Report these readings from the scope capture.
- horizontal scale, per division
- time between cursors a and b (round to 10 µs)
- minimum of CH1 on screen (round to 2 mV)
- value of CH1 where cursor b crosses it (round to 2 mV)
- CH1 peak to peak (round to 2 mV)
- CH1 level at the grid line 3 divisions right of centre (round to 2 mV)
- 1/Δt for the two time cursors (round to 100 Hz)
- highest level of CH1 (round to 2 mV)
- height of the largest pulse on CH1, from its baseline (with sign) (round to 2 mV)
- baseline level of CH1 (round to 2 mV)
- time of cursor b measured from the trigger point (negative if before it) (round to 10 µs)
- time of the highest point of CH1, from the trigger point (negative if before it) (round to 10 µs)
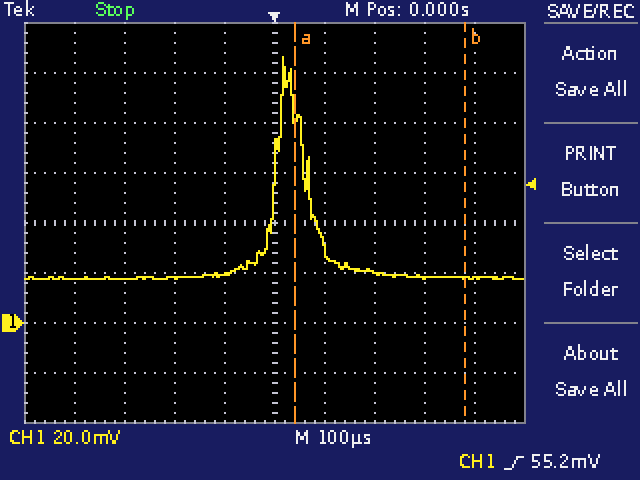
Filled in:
100 µs
340 µs
18 mV
18 mV
88 mV
18 mV
2.9 kHz
106 mV
+88 mV
18 mV
+380 µs
+20 µs
